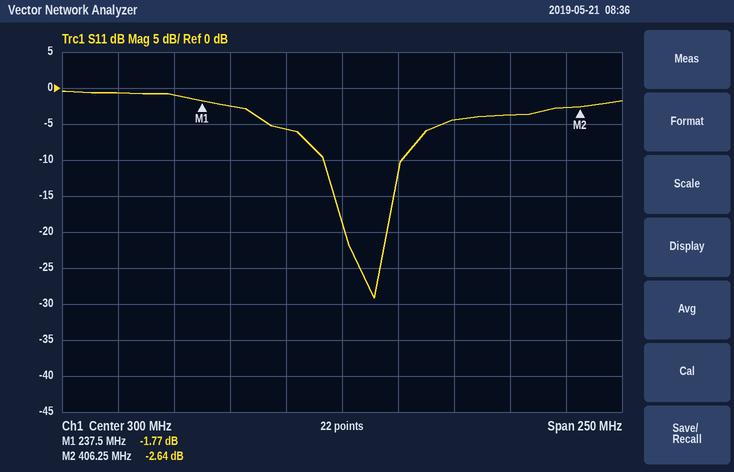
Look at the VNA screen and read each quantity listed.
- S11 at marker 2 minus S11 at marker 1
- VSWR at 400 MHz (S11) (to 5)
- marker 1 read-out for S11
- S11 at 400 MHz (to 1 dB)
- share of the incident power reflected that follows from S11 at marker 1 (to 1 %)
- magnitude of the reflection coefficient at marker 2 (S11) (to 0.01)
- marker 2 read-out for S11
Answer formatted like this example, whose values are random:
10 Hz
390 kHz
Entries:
-0.87 dB
5
-1.77 dB
-3 dB
67 %
0.74
-2.64 dB
